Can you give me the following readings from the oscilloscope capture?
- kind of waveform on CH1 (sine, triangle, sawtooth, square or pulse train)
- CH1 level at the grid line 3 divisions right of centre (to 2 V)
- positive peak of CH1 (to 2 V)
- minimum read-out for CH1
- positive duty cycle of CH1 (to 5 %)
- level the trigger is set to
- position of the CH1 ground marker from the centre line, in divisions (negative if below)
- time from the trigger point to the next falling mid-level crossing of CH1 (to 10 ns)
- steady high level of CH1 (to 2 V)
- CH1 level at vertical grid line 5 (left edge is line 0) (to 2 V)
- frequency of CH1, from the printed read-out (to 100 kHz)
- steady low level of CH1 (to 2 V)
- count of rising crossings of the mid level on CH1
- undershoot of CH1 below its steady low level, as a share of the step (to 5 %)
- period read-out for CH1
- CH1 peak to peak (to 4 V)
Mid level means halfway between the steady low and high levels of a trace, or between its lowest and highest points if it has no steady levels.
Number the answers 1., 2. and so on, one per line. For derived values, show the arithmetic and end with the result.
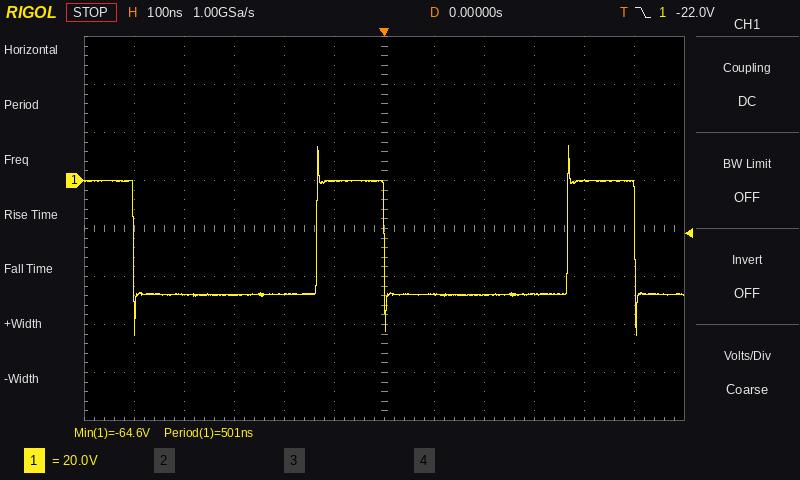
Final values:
1. pulse train
2. -48 V
3. 14 V
4. -64.6 V
5. 25 %
6. -22.0 V
7. +1.0 div
8. 500 ns
9. 0 V
10. 0 V
11. 1 / 501 ns ≈ 2.0 MHz
12. -48 V
13. 2
14. 35 %
15. 501 ns
16. 80 V
